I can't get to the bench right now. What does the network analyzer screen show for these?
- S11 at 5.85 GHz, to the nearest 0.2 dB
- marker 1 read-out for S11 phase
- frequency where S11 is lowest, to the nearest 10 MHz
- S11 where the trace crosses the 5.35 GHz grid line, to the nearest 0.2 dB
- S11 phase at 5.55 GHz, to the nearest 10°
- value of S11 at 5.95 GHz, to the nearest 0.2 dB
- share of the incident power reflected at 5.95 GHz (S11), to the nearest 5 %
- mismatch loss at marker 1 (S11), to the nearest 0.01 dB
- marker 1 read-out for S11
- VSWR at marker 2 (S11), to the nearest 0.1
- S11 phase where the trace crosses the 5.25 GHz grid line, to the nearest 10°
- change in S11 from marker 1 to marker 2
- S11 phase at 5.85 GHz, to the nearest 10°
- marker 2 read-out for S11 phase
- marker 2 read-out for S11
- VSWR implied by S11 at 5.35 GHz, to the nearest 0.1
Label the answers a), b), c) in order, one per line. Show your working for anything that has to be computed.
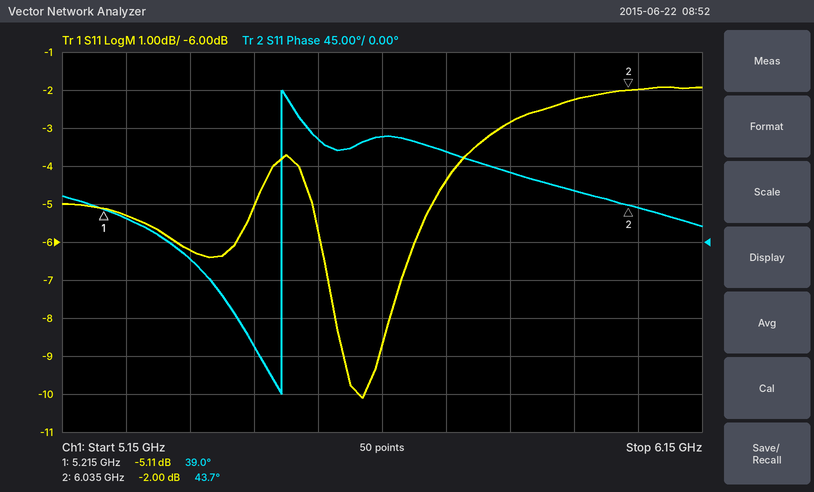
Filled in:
a) -2.8 dB
b) 39.0°
c) 5.62 GHz
d) -6.2 dB
e) 120°
f) -2.2 dB
g) 10^(-2.2/10) ≈ 60 %
h) −10 log10(1 − 10^(-5.11/10)) ≈ 1.60 dB
i) -5.11 dB
j) (1 + 0.7943)/(1 − 0.7943) ≈ 8.7
k) 30°
l) -2 − (-5.11) = 3.11 dB
m) 80°
n) 43.7°
o) -2.00 dB
p) |Γ| = 10^(-6.2/20) = 0.4898; VSWR = (1 + 0.4898)/(1 − 0.4898) ≈ 2.9
